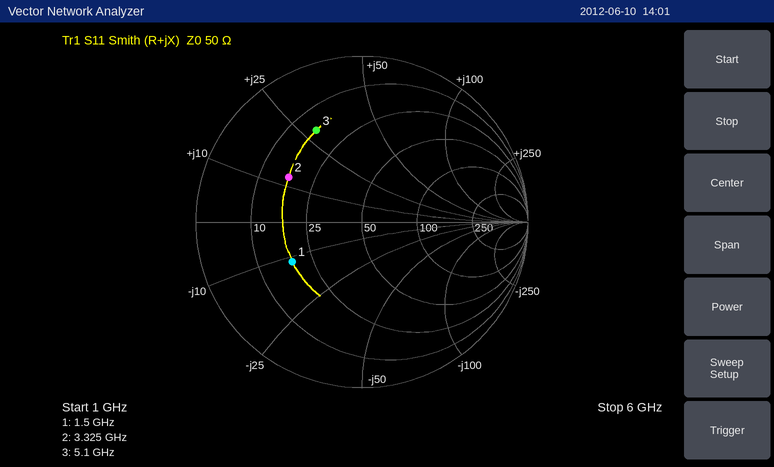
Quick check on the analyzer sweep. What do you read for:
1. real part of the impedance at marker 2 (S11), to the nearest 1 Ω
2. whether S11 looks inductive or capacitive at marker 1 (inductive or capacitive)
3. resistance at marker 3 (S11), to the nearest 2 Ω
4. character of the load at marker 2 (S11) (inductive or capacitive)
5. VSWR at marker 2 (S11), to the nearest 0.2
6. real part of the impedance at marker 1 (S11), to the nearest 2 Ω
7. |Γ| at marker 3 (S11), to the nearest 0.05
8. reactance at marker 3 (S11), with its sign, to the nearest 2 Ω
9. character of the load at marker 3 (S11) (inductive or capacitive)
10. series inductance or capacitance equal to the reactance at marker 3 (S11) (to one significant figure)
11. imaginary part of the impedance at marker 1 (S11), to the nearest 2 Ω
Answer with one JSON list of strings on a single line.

["17 Ω", "capacitive", "16 Ω", "inductive", "3.2", "18 Ω", "0.60", "+28 Ω", "inductive", "900 pH", "-12 Ω"]
